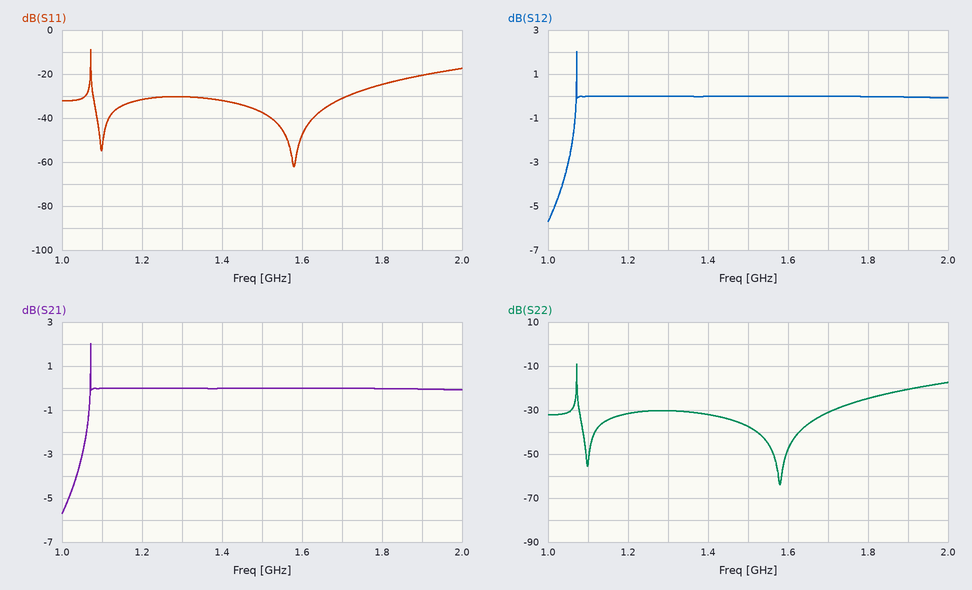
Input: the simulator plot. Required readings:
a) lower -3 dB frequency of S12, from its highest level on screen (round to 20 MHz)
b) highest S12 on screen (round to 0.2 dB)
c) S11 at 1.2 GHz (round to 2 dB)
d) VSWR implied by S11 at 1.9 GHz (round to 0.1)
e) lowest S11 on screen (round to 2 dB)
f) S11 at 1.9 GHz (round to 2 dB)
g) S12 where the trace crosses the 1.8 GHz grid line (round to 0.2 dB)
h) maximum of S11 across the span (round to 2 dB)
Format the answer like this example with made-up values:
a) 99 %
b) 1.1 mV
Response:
a) 1.06 GHz
b) 2.0 dB
c) -32 dB
d) 1.2
e) -62 dB
f) -20 dB
g) 0.0 dB
h) -8 dB
